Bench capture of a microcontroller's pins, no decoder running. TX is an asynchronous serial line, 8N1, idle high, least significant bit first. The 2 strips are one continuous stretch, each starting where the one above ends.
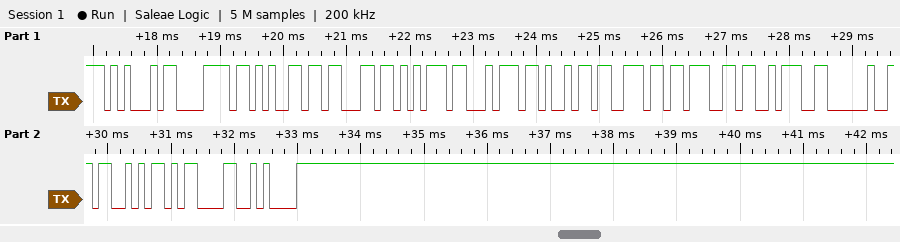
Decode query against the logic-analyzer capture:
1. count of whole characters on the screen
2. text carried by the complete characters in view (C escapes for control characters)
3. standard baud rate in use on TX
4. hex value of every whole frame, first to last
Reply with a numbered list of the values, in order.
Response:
1. 14
2. "Executing: S\r\n"
3. 9600 baud
4. 0x45 0x78 0x65 0x63 0x75 0x74 0x69 0x6E 0x67 0x3A 0x20 0x53 0x0D 0x0A
